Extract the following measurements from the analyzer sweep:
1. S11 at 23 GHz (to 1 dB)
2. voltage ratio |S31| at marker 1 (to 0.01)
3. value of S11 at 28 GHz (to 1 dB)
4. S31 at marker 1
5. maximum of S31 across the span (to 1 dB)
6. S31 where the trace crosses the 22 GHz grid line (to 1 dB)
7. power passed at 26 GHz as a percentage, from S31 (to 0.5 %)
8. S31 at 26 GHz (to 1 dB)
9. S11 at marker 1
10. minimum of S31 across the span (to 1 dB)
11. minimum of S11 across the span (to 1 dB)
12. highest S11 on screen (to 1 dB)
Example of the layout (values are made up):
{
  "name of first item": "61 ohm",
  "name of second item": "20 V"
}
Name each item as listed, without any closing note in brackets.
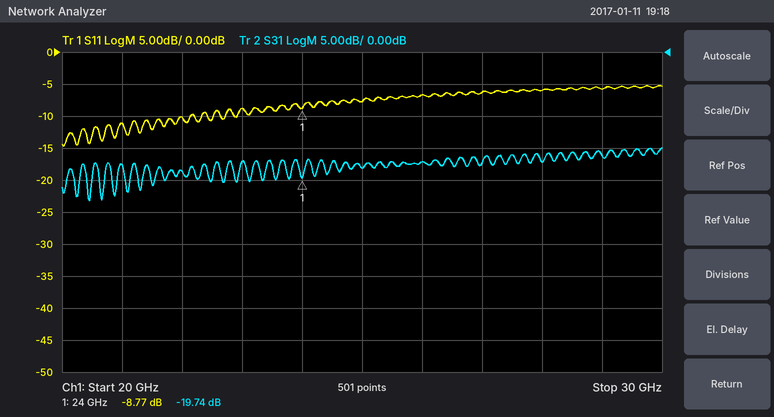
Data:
{
  "S11 at 23 GHz": "-9 dB",
  "voltage ratio |S31| at marker 1": "0.10",
  "value of S11 at 28 GHz": "-6 dB",
  "S31 at marker 1": "-19.74 dB",
  "maximum of S31 across the span": "-15 dB",
  "S31 where the trace crosses the 22 GHz grid line": "-19 dB",
  "power passed at 26 GHz as a percentage, from S31": "2.0 %",
  "S31 at 26 GHz": "-17 dB",
  "S11 at marker 1": "-8.77 dB",
  "minimum of S31 across the span": "-23 dB",
  "minimum of S11 across the span": "-15 dB",
  "highest S11 on screen": "-5 dB"
}
